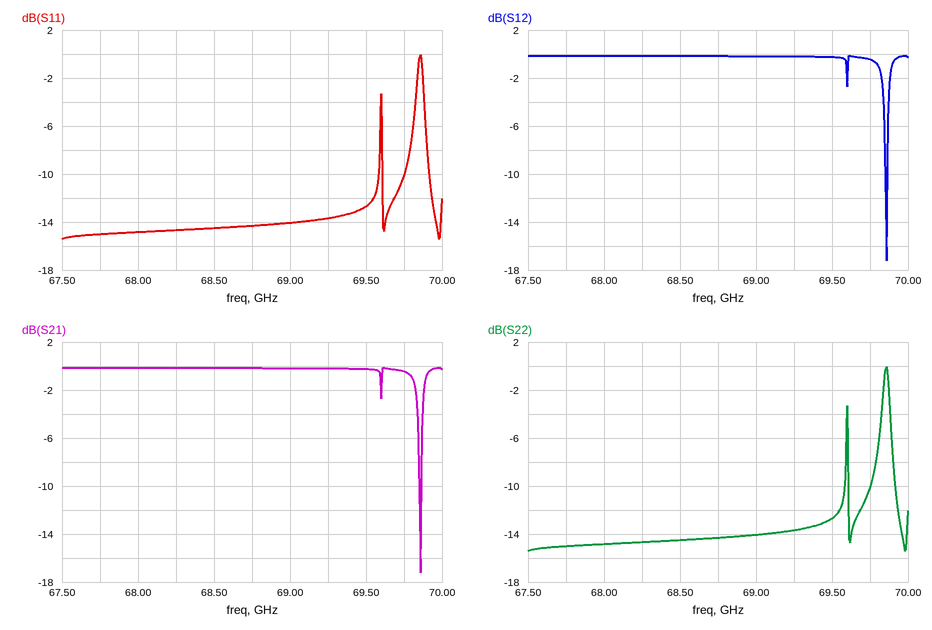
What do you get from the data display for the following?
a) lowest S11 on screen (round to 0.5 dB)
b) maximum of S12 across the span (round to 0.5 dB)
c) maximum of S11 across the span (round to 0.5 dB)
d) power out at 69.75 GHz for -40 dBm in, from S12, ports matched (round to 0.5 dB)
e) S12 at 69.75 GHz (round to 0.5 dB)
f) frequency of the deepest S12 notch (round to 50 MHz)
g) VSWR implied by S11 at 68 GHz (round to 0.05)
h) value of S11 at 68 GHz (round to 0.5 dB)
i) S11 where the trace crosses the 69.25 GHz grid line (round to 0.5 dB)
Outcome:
-15.5 dB
0.0 dB
0.0 dB
-40.5 dBm
-0.5 dB
69.85 GHz
1.45
-15.0 dB
-13.5 dB
